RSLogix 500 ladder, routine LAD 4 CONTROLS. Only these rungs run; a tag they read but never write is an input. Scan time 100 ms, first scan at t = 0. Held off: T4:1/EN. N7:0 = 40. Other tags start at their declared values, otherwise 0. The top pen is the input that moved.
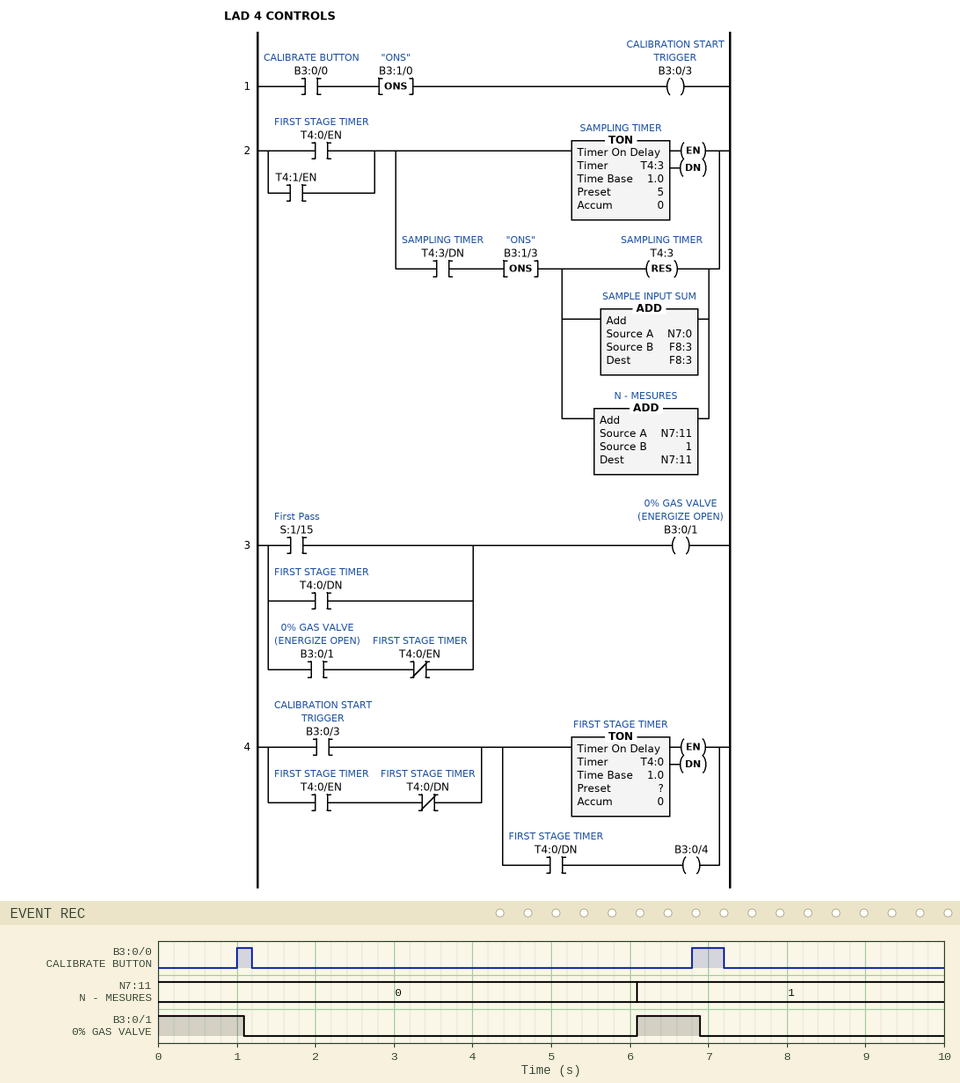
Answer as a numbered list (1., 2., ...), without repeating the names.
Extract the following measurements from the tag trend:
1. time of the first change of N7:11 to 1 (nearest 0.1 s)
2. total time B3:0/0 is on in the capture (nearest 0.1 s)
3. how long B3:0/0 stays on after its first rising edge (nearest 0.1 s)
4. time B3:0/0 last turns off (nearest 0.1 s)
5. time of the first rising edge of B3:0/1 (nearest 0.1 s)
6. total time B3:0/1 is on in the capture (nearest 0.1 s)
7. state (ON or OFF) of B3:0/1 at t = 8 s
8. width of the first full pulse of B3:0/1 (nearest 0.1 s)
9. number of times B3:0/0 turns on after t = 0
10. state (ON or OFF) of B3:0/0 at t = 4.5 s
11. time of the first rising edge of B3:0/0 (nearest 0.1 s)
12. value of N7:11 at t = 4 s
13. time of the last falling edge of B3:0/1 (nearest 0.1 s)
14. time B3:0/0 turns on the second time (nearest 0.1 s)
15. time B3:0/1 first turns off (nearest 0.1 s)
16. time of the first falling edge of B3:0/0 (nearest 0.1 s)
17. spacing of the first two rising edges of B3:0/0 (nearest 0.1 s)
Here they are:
1. 6.1 s
2. 0.6 s
3. 0.2 s
4. 7.2 s
5. 6.1 s
6. 1.9 s
7. OFF
8. 0.8 s
9. 2
10. OFF
11. 1.0 s
12. 0
13. 6.9 s
14. 6.8 s
15. 1.1 s
16. 1.2 s
17. 5.8 s
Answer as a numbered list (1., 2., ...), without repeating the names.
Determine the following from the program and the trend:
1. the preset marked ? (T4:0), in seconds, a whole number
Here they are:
1. 5 s
